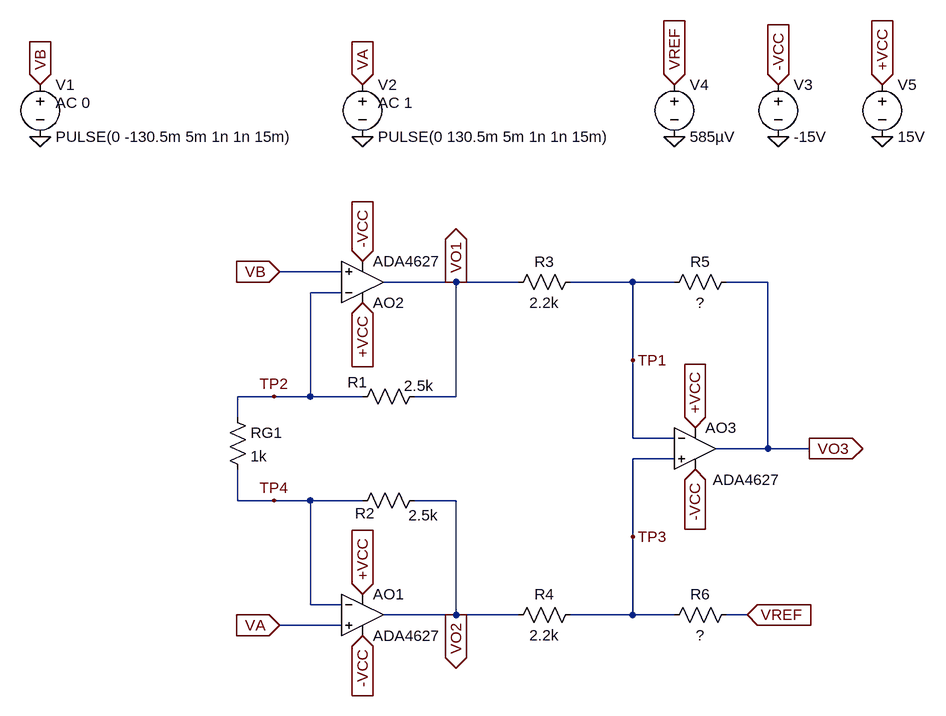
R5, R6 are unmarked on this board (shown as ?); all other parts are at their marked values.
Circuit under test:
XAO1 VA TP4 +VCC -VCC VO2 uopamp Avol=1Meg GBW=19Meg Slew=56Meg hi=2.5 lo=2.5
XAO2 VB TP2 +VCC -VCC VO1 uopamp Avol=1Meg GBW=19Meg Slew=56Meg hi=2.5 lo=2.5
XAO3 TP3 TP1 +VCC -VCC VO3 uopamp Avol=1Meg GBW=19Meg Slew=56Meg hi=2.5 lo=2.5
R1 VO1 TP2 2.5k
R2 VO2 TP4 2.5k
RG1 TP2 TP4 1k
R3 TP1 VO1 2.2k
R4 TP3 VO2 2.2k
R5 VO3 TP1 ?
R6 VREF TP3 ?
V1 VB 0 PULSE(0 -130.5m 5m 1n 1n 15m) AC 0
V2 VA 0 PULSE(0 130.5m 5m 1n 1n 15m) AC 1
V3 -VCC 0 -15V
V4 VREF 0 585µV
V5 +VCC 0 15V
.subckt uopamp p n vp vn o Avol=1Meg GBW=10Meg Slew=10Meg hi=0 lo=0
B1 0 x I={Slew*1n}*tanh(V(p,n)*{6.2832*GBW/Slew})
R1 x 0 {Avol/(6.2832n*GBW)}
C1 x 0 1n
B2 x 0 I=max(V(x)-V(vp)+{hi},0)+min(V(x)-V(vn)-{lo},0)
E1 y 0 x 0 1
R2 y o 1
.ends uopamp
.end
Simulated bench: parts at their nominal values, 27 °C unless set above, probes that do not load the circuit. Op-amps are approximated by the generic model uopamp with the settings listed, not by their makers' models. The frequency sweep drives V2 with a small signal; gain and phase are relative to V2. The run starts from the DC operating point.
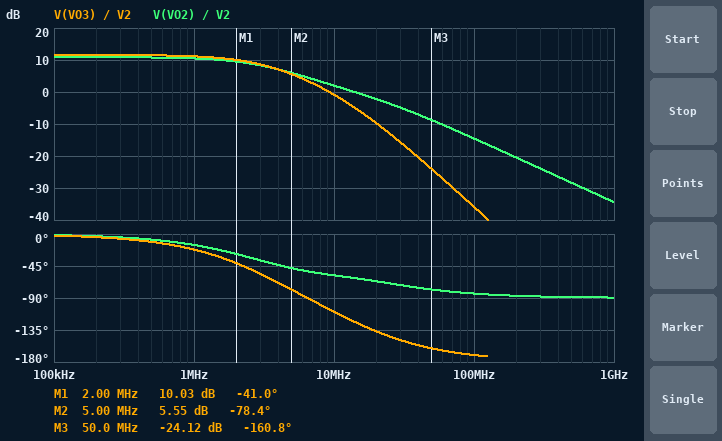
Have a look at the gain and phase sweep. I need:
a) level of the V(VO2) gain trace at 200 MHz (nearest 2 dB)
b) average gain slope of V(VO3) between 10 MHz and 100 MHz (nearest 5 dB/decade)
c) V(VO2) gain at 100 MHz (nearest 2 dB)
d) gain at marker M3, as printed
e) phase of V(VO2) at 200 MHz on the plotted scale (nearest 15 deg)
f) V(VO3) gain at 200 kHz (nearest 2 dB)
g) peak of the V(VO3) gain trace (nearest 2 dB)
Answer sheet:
-20 dB
-35 dB/decade
-14 dB
-24.12 dB
-90 deg
12 dB
12 dB
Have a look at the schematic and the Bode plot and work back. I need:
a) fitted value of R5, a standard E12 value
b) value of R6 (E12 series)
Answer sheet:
1.2 kΩ
1.8 kΩ
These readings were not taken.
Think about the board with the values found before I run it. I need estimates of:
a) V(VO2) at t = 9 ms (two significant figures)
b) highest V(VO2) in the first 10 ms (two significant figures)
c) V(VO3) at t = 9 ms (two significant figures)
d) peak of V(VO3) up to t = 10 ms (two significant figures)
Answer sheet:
780 mV
780 mV
970 mV
970 mV
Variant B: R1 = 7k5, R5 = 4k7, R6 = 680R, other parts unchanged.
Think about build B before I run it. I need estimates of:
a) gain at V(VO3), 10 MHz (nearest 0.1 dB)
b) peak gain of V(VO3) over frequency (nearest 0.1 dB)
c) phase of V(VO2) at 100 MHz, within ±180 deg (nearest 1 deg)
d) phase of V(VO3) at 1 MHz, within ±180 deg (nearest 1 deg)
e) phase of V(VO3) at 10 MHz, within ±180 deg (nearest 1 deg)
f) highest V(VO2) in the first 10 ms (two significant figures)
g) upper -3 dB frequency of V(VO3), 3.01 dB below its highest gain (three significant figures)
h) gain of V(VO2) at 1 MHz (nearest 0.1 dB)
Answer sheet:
3.5 dB
25.4 dB
-82 deg
-41 deg
-154 deg
780 mV
1.60 MHz
9.7 dB
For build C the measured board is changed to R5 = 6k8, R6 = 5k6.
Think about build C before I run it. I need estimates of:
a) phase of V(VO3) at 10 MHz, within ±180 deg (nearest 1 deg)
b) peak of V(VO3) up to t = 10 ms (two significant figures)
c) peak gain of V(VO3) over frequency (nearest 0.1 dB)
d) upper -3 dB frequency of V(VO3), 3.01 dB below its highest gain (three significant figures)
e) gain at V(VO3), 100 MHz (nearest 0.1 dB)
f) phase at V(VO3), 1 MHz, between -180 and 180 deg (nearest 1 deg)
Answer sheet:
-138 deg
4.7 V
25.1 dB
2.40 MHz
-31.7 dB
-30 deg
